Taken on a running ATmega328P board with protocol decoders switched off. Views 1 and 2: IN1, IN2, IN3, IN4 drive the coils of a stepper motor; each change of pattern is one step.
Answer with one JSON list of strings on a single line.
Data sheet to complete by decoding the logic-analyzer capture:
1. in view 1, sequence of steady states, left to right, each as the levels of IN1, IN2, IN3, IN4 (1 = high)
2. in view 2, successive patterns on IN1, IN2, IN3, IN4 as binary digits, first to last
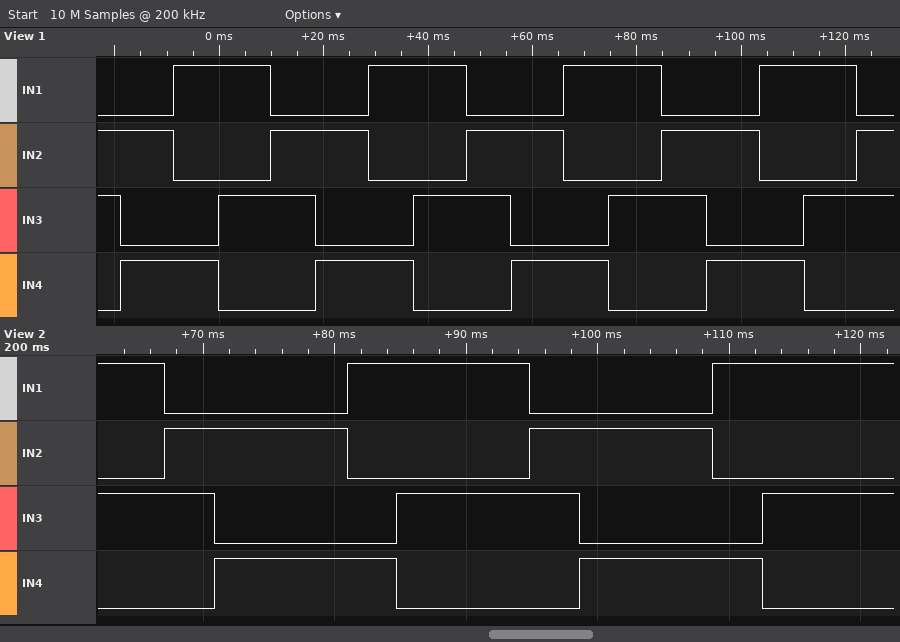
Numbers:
["0110 0101 1001 1010 0110 0101 1001 1010 0110 0101 1001 1010 0110 0101 1001 1010 0110", "1010 0110 0101 1001 1010 0110 0101 1001 1010"]
